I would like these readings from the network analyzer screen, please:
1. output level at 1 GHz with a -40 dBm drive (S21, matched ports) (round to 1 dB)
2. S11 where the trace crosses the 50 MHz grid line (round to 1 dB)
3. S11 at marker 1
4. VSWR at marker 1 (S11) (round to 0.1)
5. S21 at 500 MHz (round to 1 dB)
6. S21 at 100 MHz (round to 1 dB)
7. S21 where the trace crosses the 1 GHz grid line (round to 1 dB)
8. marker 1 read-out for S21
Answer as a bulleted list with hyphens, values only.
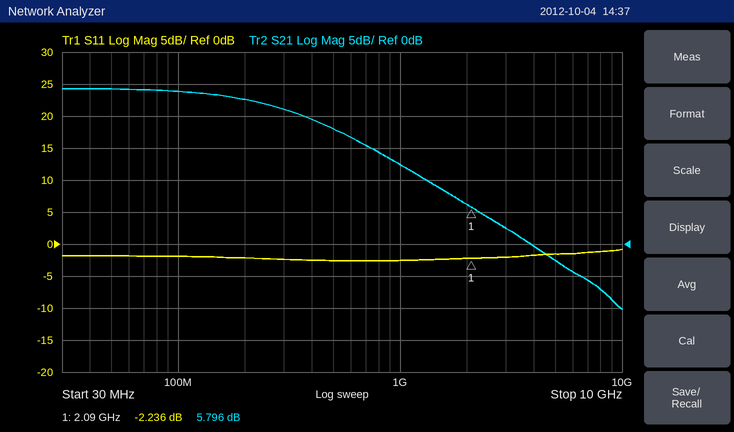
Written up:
- -28 dBm
- -2 dB
- -2.236 dB
- 7.8
- 18 dB
- 24 dB
- 12 dB
- 5.796 dB
